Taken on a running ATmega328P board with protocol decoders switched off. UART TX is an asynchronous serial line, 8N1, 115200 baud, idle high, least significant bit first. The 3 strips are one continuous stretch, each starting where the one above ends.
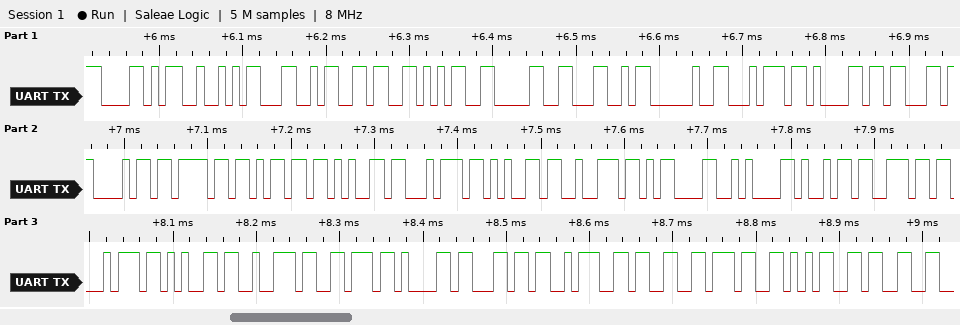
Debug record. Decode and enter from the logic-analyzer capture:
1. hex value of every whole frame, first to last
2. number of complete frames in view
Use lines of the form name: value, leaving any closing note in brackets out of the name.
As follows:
hex value of every whole frame, first to last: 58 52 4C 36 35 30 4C 20 74 61 63 68 6F 6D 65 74 65 72 0D 0A 69 6E 74 65 72 76 61 6C 3A 33 37 35 33
number of complete frames in view: 33
